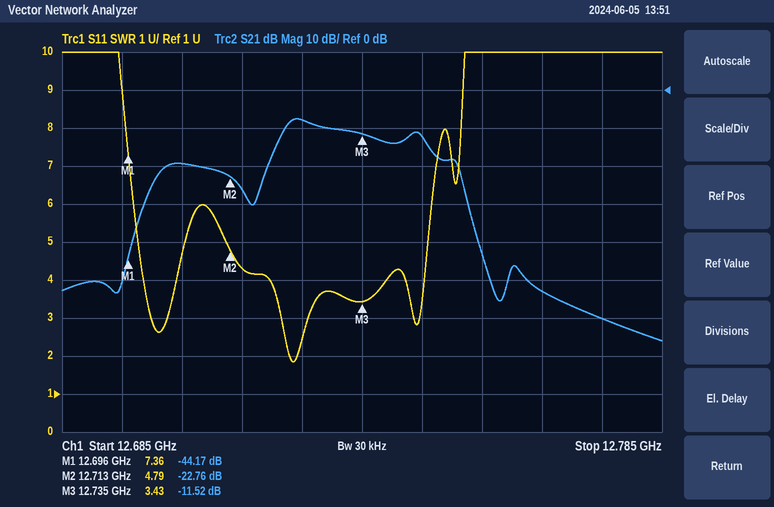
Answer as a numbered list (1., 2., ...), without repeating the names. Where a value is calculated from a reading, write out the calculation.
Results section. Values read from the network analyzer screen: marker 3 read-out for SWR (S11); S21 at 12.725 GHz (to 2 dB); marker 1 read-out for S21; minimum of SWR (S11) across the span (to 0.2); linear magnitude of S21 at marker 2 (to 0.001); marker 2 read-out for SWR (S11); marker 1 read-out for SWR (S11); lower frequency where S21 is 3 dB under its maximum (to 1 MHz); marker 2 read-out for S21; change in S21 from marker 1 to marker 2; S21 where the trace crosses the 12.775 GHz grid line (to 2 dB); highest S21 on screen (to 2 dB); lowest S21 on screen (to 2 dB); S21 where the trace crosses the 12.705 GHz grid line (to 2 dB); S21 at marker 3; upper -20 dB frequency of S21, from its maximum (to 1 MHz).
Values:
1. 3.43
2. -8 dB
3. -44.17 dB
4. 1.8
5. 10^(-22.76/20) ≈ 0.073
6. 4.79
7. 7.36
8. 12.722 GHz
9. -22.76 dB
10. -22.76 − (-44.17) = 21.41 dB
11. -60 dB
12. -8 dB
13. -66 dB
14. -20 dB
15. -11.52 dB
16. 12.752 GHz
